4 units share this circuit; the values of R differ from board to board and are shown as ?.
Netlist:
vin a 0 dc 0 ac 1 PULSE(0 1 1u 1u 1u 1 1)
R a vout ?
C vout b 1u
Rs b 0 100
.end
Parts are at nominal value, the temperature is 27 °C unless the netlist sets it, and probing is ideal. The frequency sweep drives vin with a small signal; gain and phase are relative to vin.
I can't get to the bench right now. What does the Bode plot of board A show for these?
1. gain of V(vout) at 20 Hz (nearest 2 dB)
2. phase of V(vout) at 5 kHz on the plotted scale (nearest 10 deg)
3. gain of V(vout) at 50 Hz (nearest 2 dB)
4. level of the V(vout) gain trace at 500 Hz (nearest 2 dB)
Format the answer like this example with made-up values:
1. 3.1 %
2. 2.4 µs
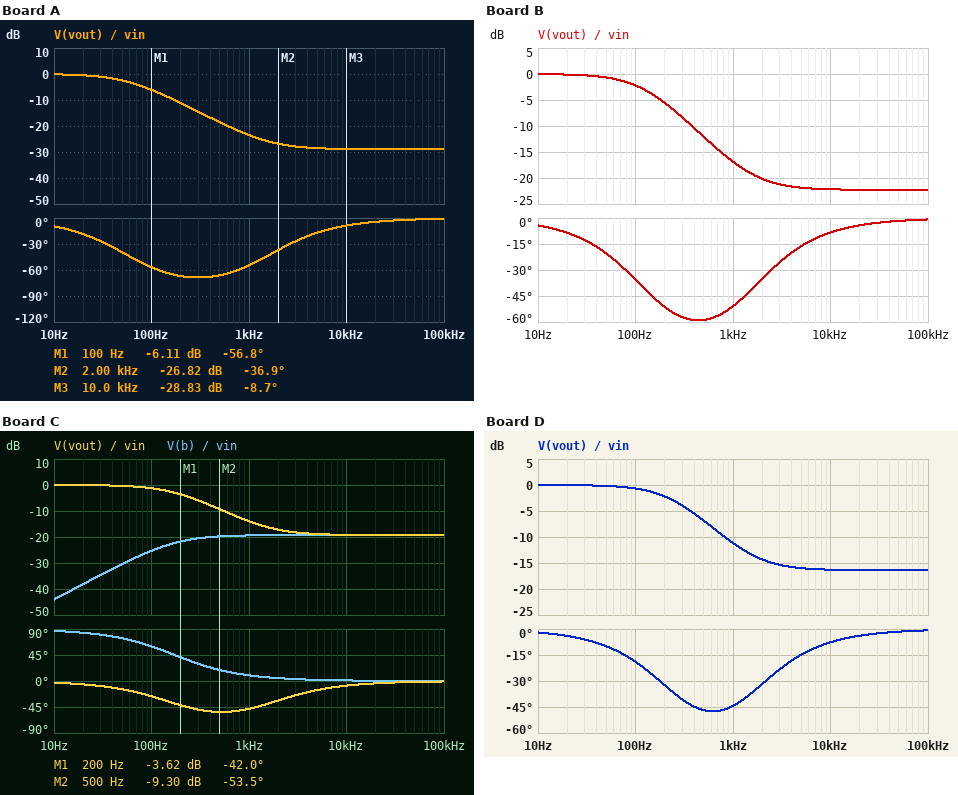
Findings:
1. 0 dB
2. -20 deg
3. -2 dB
4. -18 dB
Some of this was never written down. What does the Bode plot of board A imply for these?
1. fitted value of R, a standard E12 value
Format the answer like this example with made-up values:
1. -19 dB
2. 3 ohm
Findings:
1. 2.7 kΩ
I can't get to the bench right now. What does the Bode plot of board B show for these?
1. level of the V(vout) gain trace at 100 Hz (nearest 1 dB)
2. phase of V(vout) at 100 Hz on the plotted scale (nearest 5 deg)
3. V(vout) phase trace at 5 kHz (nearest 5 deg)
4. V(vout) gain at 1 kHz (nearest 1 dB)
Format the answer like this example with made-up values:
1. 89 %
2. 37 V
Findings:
1. -2 dB
2. -35 deg
3. -15 deg
4. -17 dB
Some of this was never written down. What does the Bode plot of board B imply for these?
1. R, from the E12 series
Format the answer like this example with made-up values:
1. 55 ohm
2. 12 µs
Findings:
1. 1.2 kΩ
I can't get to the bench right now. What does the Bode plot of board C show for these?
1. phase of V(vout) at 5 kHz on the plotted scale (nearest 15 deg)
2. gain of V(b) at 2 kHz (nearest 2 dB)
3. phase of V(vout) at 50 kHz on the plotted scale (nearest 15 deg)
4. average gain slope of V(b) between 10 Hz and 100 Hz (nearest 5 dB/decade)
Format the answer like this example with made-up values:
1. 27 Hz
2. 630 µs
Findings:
1. -15 deg
2. -20 dB
3. 0 deg
4. 20 dB/decade
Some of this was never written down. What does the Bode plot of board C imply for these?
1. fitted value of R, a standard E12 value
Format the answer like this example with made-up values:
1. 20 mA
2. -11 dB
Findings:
1. 820 Ω
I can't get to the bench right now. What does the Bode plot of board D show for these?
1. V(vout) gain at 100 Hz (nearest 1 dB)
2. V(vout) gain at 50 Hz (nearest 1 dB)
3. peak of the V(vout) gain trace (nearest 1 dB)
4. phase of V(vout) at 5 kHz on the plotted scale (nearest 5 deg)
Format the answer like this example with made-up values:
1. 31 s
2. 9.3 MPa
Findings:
1. -1 dB
2. 0 dB
3. 0 dB
4. -15 deg
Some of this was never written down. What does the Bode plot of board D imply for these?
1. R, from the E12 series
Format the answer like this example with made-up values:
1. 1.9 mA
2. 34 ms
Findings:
1. 560 Ω
